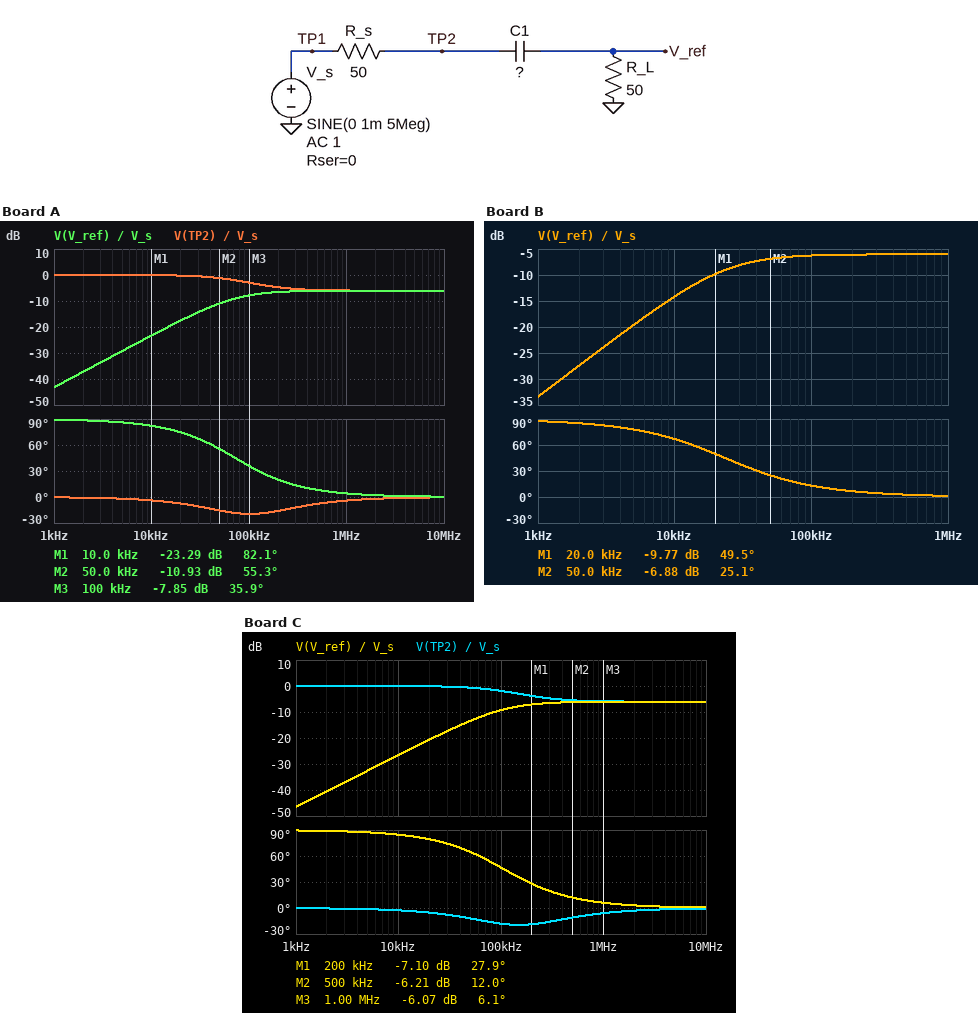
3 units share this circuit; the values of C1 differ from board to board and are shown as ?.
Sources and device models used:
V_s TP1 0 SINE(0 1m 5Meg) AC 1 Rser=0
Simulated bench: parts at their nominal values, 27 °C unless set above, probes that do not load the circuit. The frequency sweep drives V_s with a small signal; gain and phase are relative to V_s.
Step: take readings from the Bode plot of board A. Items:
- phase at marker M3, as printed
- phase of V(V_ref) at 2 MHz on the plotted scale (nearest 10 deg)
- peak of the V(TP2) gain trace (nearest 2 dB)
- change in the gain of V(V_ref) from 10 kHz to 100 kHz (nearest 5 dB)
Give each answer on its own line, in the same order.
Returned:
35.9 deg
0 deg
0 dB
15 dB
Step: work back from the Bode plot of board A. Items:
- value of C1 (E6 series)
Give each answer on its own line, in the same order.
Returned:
22 nF
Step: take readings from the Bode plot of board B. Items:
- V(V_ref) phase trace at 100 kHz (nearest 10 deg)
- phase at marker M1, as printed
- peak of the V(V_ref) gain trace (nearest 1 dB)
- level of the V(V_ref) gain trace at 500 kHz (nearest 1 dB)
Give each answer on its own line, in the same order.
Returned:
10 deg
49.5 deg
-6 dB
-6 dB
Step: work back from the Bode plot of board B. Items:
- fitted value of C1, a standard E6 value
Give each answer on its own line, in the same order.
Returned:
68 nF
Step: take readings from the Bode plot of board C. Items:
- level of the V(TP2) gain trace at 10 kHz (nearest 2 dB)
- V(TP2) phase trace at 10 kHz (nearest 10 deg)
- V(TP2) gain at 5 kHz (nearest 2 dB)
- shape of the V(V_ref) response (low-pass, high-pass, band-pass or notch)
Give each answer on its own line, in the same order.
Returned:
0 dB
0 deg
0 dB
high-pass
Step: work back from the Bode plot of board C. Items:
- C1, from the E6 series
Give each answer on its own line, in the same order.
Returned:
15 nF
